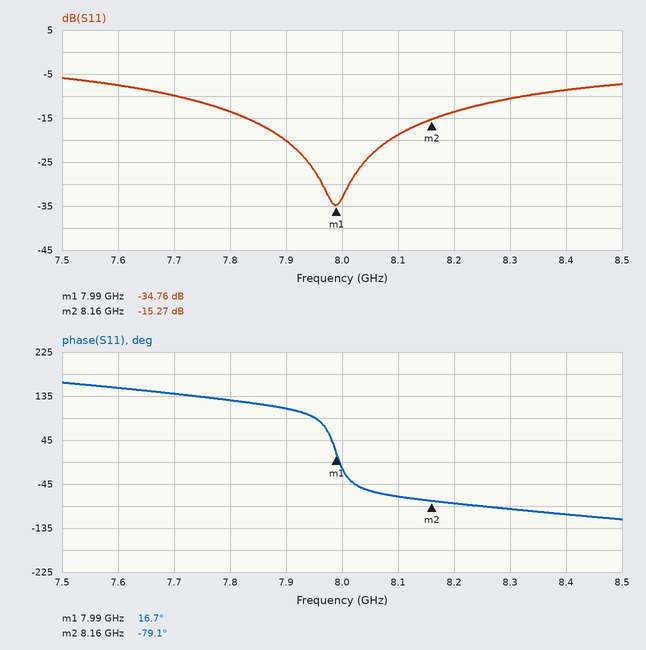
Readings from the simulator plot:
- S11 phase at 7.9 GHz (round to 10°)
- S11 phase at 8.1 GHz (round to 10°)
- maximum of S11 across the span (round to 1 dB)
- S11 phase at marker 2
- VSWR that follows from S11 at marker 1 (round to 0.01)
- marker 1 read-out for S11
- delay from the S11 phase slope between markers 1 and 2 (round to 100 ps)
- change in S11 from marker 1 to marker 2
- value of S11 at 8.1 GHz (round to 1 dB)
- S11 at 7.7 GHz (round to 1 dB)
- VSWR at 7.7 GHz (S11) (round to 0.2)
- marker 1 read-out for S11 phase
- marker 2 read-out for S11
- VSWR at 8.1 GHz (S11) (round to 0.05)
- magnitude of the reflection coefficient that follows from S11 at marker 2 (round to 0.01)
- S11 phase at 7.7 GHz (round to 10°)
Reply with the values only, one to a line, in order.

110°
-70°
-6 dB
-79.1°
1.04
-34.76 dB
1.6 ns
19.49 dB
-19 dB
-10 dB
2.0
16.7°
-15.27 dB
1.25
0.17
140°
